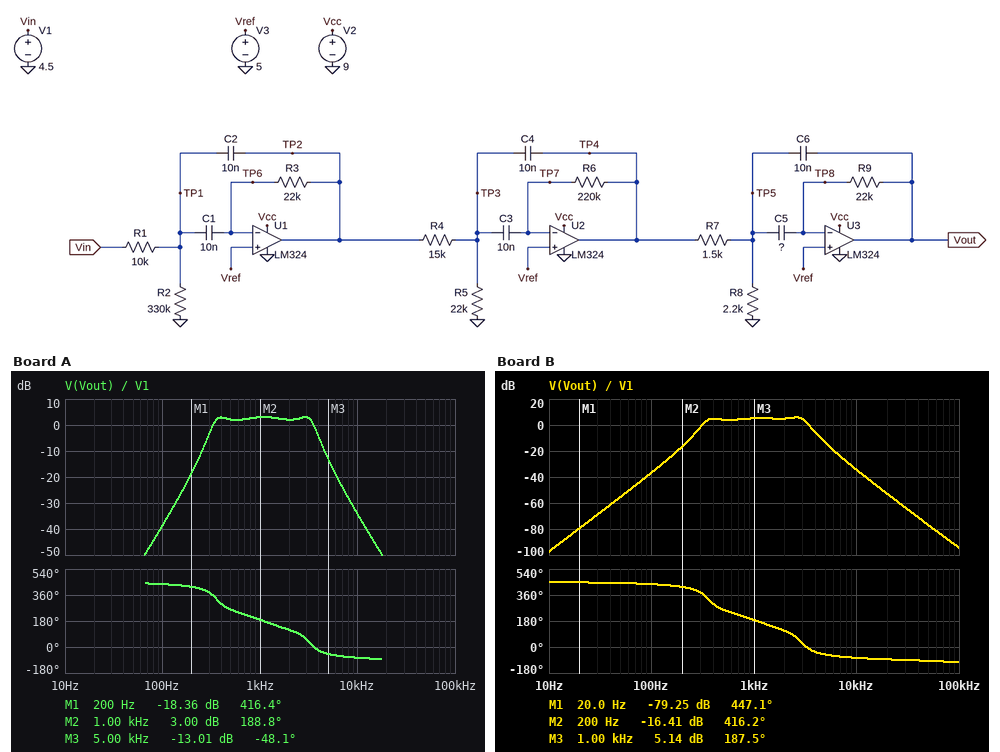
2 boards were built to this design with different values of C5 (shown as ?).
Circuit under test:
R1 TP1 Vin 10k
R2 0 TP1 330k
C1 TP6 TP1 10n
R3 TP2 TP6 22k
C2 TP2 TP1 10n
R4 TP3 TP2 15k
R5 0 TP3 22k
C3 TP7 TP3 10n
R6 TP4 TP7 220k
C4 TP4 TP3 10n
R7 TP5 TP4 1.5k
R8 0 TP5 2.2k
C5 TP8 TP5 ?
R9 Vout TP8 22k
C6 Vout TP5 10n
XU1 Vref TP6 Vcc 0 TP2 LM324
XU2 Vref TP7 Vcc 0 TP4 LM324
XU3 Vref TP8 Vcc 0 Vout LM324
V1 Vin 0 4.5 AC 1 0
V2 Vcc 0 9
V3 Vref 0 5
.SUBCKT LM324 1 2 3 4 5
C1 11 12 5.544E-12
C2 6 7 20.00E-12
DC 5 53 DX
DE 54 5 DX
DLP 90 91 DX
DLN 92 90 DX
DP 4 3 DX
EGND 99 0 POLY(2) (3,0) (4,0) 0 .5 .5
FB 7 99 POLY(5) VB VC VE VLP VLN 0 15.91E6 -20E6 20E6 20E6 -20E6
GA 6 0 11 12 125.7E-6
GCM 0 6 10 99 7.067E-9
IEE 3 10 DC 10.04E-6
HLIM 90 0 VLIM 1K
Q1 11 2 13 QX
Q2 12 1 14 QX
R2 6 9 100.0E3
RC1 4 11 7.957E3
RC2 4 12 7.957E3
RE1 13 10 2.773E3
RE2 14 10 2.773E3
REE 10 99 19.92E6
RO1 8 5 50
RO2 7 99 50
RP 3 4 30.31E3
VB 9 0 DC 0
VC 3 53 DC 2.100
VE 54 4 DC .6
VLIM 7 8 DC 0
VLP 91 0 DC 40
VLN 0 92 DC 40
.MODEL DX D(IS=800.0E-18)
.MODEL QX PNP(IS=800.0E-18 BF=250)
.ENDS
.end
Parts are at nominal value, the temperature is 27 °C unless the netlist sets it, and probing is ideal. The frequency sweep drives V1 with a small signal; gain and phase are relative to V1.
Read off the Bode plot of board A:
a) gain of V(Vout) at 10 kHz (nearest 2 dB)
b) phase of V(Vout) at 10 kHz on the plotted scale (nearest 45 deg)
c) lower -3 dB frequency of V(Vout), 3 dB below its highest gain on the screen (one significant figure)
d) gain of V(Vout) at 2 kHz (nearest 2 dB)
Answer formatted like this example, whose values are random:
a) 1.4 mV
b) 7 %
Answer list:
a) -34 dB
b) -90 deg
c) 300 Hz
d) 2 dB
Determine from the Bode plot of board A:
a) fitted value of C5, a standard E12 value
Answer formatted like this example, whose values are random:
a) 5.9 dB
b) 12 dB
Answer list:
a) 12 nF
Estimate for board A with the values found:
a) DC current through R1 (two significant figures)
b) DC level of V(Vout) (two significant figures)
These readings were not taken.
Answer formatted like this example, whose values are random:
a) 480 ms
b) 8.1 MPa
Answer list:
a) 13 µA
b) 5.0 V
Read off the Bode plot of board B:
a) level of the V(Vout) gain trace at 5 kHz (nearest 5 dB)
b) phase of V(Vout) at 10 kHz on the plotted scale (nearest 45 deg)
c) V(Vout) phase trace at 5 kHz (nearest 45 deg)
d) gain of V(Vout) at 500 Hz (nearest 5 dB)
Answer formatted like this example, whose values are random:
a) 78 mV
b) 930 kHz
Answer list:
a) -15 dB
b) -90 deg
c) -45 deg
d) 5 dB
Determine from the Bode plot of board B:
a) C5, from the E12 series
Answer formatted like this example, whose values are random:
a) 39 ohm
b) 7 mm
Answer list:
a) 15 nF
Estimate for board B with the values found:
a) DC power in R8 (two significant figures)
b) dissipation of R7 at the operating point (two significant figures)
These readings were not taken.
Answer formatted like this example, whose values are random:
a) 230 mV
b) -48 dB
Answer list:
a) 4.0 mW
b) 2.7 mW
